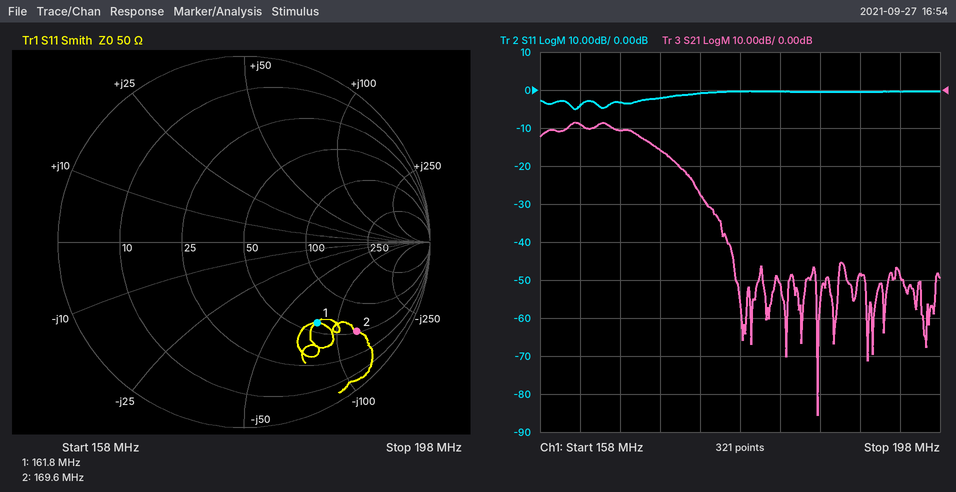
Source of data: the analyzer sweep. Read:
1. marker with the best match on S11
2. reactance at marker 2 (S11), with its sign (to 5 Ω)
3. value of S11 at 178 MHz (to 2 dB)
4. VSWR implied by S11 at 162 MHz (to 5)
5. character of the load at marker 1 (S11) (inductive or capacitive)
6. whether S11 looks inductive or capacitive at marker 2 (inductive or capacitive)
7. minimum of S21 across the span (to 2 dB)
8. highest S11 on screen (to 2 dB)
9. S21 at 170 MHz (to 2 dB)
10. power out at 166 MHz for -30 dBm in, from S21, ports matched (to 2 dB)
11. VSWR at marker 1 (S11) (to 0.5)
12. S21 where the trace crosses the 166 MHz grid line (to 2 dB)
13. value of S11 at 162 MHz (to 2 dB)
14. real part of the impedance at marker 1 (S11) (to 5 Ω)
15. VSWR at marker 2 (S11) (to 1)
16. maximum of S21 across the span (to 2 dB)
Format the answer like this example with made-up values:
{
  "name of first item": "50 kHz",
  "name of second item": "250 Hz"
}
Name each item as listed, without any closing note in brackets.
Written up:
{
  "marker with the best match on S11": "marker 1",
  "reactance at marker 2 (S11), with its sign": "-125 Ω",
  "value of S11 at 178 MHz": "0 dB",
  "VSWR implied by S11 at 162 MHz": "5",
  "character of the load at marker 1 (S11)": "capacitive",
  "whether S11 looks inductive or capacitive at marker 2": "capacitive",
  "minimum of S21 across the span": "-86 dB",
  "highest S11 on screen": "0 dB",
  "S21 at 170 MHz": "-16 dB",
  "power out at 166 MHz for -30 dBm in, from S21, ports matched": "-40 dBm",
  "VSWR at marker 1 (S11)": "4.0",
  "S21 where the trace crosses the 166 MHz grid line": "-10 dB",
  "value of S11 at 162 MHz": "-4 dB",
  "real part of the impedance at marker 1 (S11)": "60 Ω",
  "VSWR at marker 2 (S11)": "8",
  "maximum of S21 across the span": "-8 dB"
}
